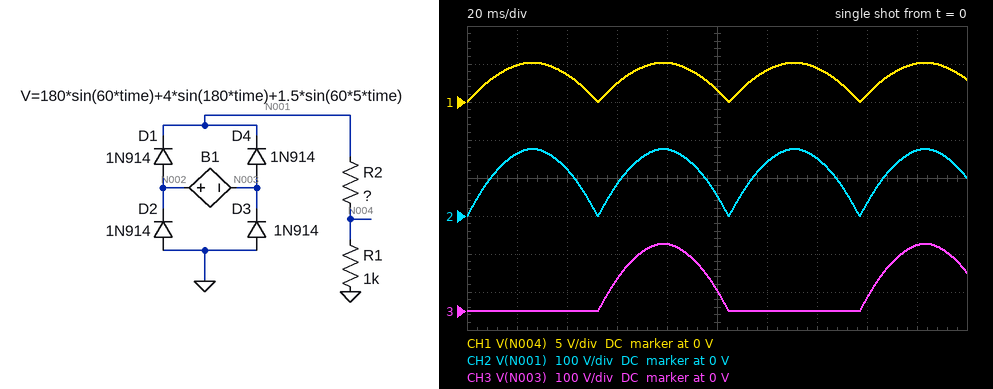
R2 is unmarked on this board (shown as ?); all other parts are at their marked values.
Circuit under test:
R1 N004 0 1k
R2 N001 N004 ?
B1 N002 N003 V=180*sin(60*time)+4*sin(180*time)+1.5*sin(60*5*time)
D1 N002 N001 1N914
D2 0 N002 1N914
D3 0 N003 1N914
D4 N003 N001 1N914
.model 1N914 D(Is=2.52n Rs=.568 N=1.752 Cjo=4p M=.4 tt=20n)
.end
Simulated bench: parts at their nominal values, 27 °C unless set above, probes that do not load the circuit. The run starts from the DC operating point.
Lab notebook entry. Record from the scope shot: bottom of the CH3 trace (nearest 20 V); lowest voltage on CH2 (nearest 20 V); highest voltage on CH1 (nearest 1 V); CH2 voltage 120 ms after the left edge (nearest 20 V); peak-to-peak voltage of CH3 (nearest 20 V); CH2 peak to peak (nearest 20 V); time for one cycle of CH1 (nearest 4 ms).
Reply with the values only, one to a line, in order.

0 V
0 V
5 V
140 V
180 V
180 V
52 ms
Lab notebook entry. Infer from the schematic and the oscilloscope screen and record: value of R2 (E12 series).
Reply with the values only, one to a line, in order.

33 kΩ
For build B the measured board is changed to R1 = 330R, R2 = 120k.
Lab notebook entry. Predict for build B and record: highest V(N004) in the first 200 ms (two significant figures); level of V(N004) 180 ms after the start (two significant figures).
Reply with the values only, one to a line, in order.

480 mV
470 mV
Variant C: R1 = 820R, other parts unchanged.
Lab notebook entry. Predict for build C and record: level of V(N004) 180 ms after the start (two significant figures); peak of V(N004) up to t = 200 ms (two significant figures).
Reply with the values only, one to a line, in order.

4.2 V
4.3 V
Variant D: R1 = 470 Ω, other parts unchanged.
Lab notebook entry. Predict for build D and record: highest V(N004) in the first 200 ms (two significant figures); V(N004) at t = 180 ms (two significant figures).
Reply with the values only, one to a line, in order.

2.5 V
2.4 V
